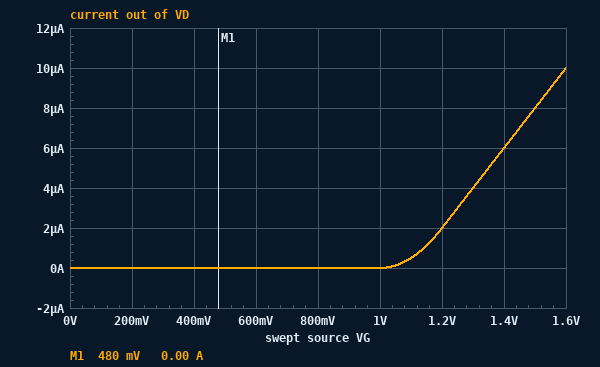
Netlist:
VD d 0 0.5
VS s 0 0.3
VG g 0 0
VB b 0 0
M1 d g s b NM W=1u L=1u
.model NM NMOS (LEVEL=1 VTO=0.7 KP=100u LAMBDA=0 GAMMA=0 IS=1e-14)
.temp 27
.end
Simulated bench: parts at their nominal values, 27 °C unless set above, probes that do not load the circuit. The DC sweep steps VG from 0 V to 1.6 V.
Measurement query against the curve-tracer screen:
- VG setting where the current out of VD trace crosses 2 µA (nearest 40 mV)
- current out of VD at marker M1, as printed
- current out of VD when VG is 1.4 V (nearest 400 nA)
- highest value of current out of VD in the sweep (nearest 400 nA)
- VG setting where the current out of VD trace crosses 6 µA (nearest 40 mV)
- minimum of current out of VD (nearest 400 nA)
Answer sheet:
1.20 V
0.00 A
6.0 µA
10.0 µA
1.40 V
0 A
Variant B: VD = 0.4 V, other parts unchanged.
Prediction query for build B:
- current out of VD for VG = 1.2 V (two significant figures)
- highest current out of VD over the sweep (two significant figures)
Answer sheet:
1.5 µA
5.5 µA
